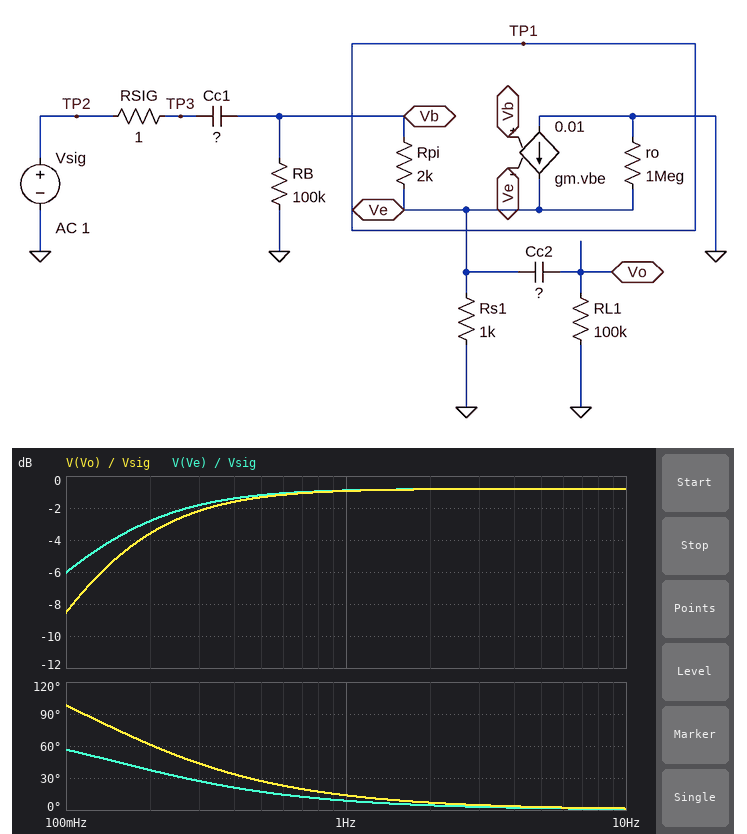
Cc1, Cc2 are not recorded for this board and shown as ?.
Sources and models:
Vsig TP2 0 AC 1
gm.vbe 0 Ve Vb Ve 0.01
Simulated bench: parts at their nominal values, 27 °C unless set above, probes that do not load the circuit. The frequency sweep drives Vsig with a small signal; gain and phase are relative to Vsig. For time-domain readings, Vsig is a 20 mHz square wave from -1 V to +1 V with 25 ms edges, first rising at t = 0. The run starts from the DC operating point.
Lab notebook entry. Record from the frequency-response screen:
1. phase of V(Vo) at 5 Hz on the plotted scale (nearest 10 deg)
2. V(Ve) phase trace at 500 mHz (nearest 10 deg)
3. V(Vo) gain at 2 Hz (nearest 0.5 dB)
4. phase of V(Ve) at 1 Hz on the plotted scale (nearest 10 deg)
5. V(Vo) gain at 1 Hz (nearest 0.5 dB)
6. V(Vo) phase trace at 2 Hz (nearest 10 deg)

0 deg
20 deg
-1.0 dB
10 deg
-1.0 dB
10 deg
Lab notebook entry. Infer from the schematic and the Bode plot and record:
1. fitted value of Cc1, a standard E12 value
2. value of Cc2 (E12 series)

56 µF
18 µF
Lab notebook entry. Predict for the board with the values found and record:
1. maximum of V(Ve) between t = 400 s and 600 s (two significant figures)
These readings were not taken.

1.8 V
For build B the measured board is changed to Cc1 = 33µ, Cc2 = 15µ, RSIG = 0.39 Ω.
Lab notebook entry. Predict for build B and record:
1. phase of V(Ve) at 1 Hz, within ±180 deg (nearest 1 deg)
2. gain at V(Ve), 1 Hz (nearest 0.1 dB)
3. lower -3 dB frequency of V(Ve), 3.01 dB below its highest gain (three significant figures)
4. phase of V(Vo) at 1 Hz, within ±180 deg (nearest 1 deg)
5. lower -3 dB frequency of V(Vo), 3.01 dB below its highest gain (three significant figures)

15 deg
-1.1 dB
260 mHz
21 deg
296 mHz
